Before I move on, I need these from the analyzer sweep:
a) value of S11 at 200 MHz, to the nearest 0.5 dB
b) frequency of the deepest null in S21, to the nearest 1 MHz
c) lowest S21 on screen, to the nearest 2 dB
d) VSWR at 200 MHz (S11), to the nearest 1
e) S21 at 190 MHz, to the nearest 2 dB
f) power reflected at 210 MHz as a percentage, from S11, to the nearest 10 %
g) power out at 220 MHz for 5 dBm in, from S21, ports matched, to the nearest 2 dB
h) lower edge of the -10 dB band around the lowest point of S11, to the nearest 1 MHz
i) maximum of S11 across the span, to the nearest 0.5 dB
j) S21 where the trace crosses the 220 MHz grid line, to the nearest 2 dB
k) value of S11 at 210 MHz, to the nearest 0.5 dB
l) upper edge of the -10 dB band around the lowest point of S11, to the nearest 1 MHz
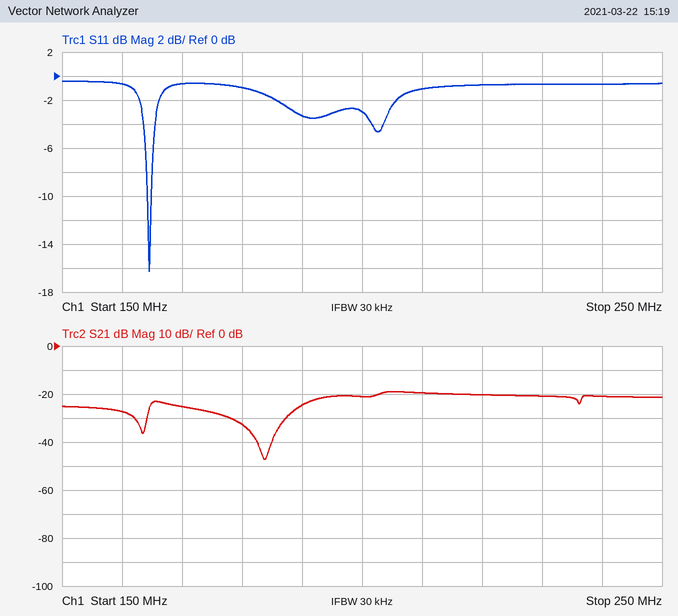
-3.0 dB
184 MHz
-48 dB
6
-24 dB
80 %
-16 dBm
164 MHz
-0.5 dB
-20 dB
-1.0 dB
165 MHz
